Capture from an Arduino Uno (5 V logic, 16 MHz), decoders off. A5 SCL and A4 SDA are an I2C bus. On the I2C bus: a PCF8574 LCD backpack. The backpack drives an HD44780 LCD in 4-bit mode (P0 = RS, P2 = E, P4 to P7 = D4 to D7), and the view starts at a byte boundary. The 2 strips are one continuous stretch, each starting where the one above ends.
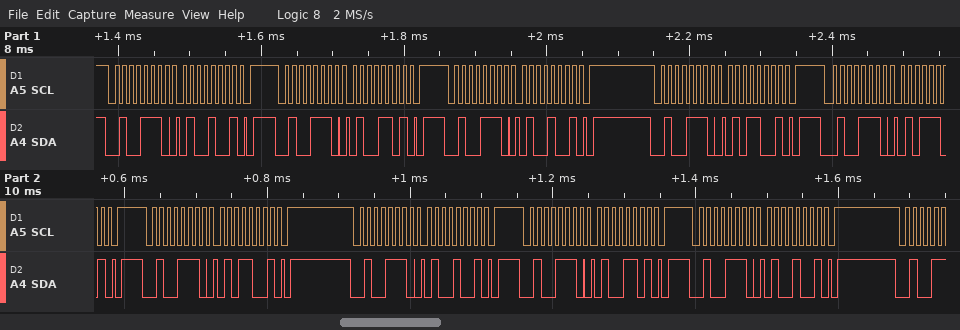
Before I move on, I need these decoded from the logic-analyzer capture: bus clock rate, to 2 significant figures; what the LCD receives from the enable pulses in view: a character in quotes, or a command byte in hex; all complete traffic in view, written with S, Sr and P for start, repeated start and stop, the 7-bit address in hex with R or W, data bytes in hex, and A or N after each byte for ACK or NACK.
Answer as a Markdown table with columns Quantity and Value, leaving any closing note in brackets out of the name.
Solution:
| Quantity | Value |
|---|---|
| bus clock rate, to 2 significant figures | 100 kHz |
| what the LCD receives from the enable pulses in view: a character in quotes, or a command byte in hex | 'E' |
| all complete traffic in view, written with S, Sr and P for start, repeated start and stop, the 7-bit address in hex with R or W, data bytes in hex, and A or N after each byte for ACK or NACK | S 27W A 49 A P S 27W A 4D A P S 27W A 49 A P S 27W A 59 A P S 27W A 5D A P S 27W A 59 A P S 27W A 49 A P S 27W A 4D A P S 27W A 49 A P |
